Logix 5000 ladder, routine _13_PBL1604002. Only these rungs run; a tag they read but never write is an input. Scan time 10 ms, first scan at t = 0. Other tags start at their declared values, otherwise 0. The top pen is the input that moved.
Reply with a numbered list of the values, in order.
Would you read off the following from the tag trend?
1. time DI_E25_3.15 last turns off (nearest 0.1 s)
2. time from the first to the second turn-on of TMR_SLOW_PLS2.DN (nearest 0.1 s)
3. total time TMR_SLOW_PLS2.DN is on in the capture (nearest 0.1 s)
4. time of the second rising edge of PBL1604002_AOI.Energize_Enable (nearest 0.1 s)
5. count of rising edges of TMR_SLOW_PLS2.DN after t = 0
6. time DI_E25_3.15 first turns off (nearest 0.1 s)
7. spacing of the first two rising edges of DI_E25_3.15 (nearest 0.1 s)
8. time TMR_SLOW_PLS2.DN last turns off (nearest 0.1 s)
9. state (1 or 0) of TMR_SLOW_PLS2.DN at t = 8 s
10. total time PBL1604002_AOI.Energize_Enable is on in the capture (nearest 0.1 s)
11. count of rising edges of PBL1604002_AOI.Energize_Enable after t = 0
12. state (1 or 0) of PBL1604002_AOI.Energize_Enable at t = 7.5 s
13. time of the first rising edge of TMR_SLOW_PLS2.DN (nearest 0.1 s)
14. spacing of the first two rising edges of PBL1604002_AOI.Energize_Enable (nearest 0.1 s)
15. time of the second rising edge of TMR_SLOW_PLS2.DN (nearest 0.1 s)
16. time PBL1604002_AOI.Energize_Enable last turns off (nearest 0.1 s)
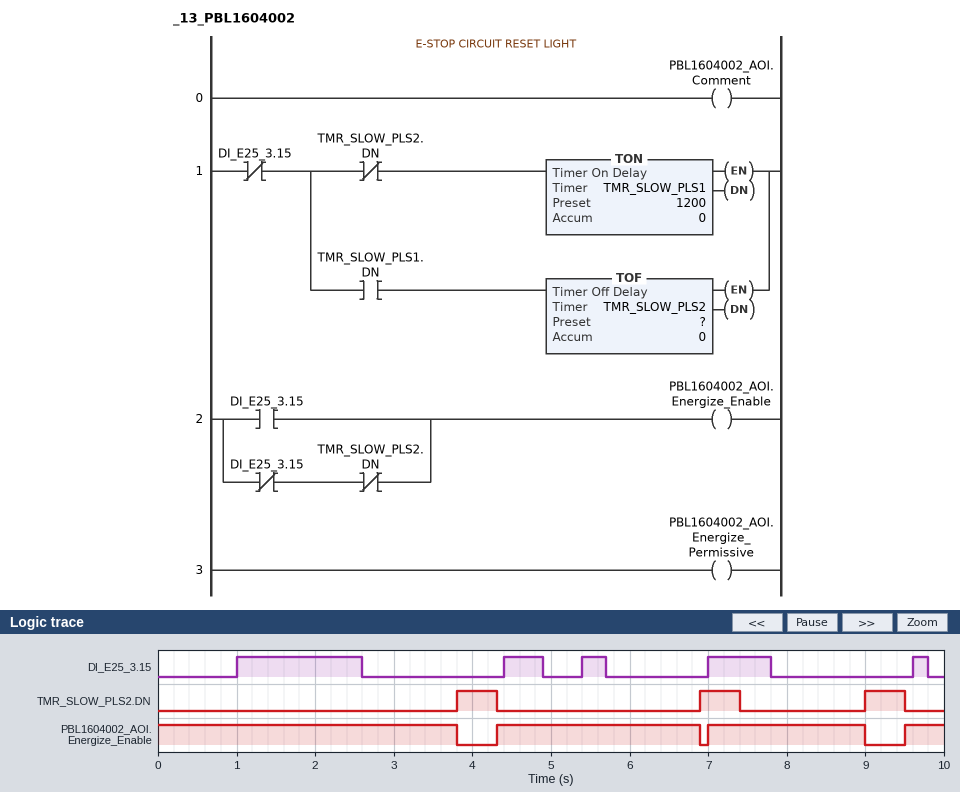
1. 9.8 s
2. 3.1 s
3. 1.5 s
4. 7.0 s
5. 3
6. 2.6 s
7. 3.4 s
8. 9.5 s
9. 0
10. 8.9 s
11. 3
12. 1
13. 3.8 s
14. 2.7 s
15. 6.9 s
16. 9.0 s
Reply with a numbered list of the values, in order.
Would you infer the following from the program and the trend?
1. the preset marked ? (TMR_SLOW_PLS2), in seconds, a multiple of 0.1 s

1. 0.5 s
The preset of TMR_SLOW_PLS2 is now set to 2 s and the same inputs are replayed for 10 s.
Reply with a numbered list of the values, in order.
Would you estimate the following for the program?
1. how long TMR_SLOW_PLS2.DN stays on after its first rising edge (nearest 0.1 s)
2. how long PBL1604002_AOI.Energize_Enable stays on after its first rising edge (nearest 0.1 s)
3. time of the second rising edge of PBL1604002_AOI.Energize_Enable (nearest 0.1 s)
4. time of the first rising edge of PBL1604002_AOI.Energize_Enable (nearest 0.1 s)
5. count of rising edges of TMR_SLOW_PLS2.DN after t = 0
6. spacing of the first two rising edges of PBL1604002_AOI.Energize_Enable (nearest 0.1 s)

1. 2.0 s
2. 0.5 s
3. 5.4 s
4. 4.4 s
5. 2
6. 1.0 s
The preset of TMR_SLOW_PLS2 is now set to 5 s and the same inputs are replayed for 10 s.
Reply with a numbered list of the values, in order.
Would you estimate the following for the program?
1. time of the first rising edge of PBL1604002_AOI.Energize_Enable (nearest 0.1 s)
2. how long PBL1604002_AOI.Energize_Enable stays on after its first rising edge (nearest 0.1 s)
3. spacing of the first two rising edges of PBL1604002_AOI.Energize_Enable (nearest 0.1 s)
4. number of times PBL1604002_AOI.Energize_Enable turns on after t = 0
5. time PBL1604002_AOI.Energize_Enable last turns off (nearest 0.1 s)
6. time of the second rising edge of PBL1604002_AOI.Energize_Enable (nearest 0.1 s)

1. 4.4 s
2. 0.5 s
3. 1.0 s
4. 4
5. 7.8 s
6. 5.4 s
